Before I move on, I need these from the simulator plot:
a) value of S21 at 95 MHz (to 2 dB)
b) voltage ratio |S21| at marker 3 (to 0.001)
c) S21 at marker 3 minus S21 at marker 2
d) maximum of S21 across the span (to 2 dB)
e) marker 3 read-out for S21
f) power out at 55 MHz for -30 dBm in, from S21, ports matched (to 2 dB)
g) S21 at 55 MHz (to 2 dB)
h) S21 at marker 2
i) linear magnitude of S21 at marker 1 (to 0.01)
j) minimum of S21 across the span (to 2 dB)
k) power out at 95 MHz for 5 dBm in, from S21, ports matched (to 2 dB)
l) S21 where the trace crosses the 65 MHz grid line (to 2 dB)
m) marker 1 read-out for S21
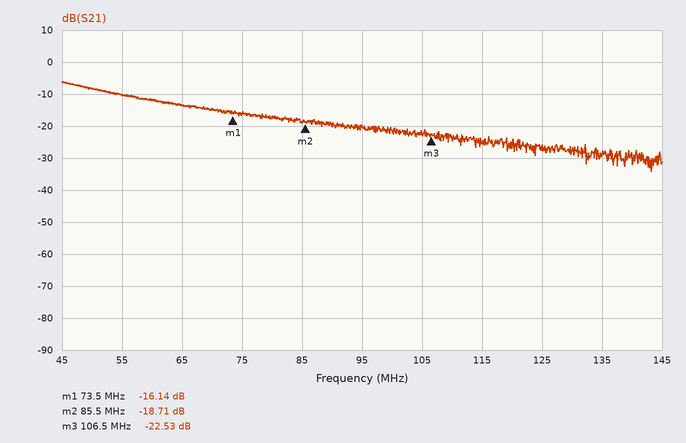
-20 dB
0.075
-3.82 dB
-6 dB
-22.53 dB
-40 dBm
-10 dB
-18.71 dB
0.16
-34 dB
-16 dBm
-14 dB
-16.14 dB
